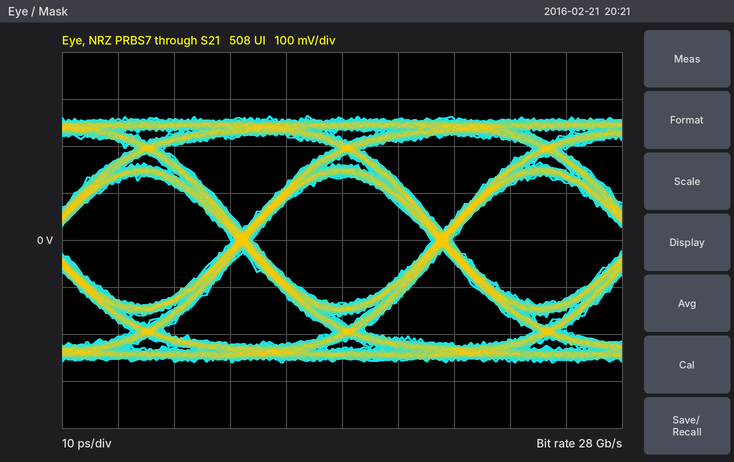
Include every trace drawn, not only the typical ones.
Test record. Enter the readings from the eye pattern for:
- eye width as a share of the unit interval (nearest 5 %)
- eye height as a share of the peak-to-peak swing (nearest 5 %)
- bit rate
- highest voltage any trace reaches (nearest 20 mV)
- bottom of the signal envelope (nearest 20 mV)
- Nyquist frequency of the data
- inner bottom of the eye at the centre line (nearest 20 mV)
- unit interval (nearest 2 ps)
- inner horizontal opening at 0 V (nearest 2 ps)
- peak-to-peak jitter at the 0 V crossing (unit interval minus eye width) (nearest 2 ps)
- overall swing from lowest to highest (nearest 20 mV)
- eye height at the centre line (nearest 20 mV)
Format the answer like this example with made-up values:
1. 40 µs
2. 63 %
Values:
1. 90 %
2. 50 %
3. 28 Gb/s
4. 260 mV
5. -260 mV
6. 14 GHz
7. -140 mV
8. 36 ps
9. 32 ps
10. 4 ps
11. 520 mV
12. 260 mV
